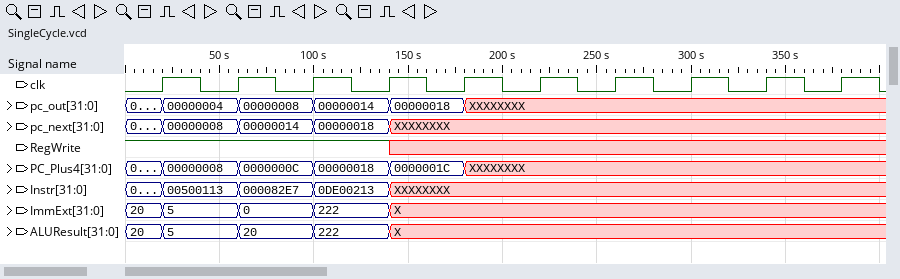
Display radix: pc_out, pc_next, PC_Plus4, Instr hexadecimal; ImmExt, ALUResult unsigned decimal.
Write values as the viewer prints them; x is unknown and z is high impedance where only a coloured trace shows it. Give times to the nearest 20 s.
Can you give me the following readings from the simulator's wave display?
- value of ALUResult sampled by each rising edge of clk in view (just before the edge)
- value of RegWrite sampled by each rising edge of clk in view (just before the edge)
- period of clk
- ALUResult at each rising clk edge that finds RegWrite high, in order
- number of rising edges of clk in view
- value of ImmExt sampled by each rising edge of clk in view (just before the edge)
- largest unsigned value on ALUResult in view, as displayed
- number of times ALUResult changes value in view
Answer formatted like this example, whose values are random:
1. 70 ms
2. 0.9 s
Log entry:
1. 20, 5, 20, 222, X, X, X, X, X, X
2. 1 1 1 1 x x x x x x
3. 40 s
4. 20, 5, 20, 222
5. 10
6. 20, 5, 0, 222, X, X, X, X, X, X
7. 222
8. 4
